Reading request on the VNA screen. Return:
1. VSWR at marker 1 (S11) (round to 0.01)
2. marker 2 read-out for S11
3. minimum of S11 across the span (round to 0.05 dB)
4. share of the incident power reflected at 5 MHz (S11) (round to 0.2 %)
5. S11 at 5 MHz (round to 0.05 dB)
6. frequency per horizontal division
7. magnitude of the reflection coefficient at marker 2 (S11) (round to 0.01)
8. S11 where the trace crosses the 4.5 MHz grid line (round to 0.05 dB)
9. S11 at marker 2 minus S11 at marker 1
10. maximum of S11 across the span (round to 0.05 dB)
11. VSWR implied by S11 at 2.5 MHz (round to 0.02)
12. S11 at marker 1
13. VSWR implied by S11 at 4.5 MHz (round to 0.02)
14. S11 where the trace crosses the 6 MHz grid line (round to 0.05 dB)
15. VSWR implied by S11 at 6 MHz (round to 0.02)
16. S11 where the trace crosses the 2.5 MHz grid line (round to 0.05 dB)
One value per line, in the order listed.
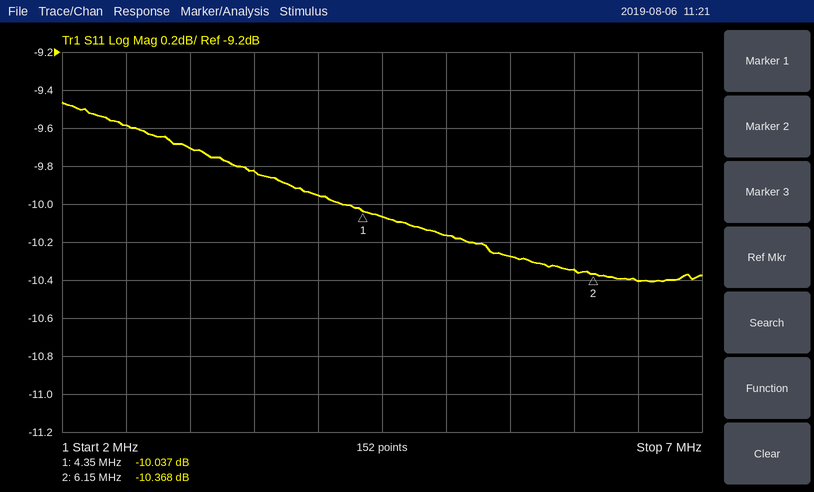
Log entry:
1.92
-10.368 dB
-10.40 dB
9.6 %
-10.15 dB
500 kHz
0.30
-10.05 dB
-0.331 dB
-9.45 dB
2.00
-10.037 dB
1.92
-10.35 dB
1.88
-9.60 dB
